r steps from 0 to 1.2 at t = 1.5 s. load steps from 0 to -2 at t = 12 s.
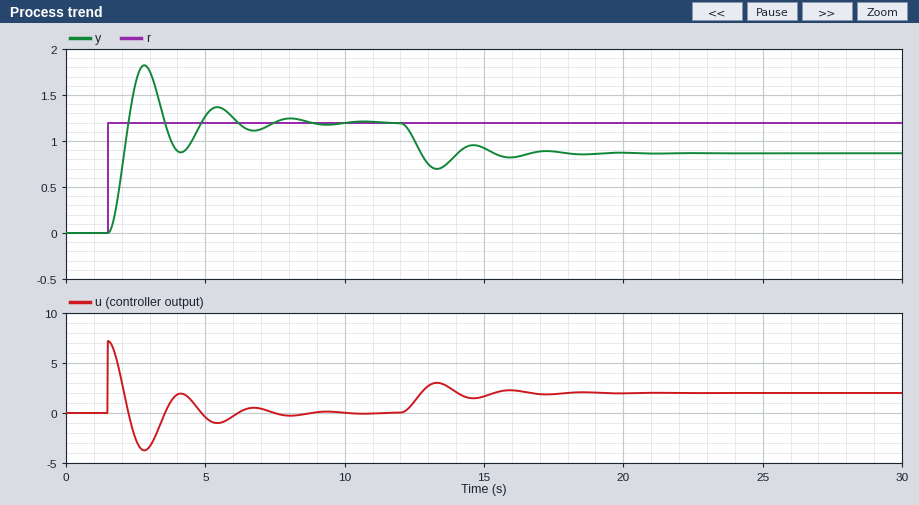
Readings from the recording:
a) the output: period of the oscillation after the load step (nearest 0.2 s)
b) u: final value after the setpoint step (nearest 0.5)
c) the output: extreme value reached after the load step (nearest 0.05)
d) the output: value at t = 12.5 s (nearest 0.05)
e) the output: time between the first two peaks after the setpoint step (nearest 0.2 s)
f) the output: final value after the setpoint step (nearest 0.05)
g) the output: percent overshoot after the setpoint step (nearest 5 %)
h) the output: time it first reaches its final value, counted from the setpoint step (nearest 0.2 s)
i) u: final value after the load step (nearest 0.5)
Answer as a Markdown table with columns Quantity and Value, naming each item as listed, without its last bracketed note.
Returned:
| Quantity | Value |
|---|---|
| the output: period of the oscillation after the load step | 2.6 s |
| u: final value after the setpoint step | 0.0 |
| the output: extreme value reached after the load step | 0.70 |
| the output: value at t = 12.5 s | 1.00 |
| the output: time between the first two peaks after the setpoint step | 2.6 s |
| the output: final value after the setpoint step | 1.20 |
| the output: percent overshoot after the setpoint step | 50 % |
| the output: time it first reaches its final value, counted from the setpoint step | 0.8 s |
| u: final value after the load step | 2.0 |
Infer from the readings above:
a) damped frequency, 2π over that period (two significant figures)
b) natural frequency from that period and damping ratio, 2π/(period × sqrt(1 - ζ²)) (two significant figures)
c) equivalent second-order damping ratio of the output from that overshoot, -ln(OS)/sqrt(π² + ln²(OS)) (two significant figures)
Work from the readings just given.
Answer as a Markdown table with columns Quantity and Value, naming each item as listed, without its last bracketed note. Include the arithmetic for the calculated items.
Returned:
| Quantity | Value |
|---|---|
| damped frequency, 2π over that period | 2π / 2.6 = 2.4 rad/s |
| natural frequency from that period and damping ratio, 2π/(period × sqrt(1 - ζ²)) | 2π / (2.6 × sqrt(1 - 0.22²)) = 2.5 rad/s |
| equivalent second-order damping ratio of the output from that overshoot, -ln(OS)/sqrt(π² + ln²(OS)) | ln(0.5) = -0.693; 0.693 / sqrt(9.870 + 0.480) = 0.22 |
